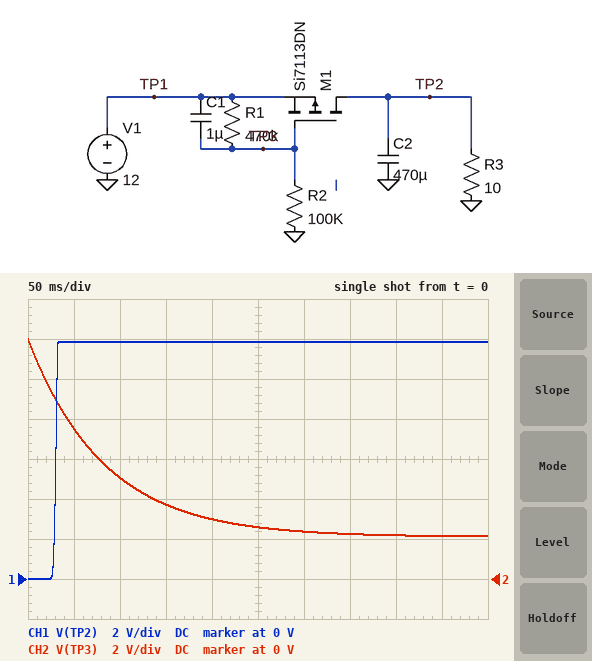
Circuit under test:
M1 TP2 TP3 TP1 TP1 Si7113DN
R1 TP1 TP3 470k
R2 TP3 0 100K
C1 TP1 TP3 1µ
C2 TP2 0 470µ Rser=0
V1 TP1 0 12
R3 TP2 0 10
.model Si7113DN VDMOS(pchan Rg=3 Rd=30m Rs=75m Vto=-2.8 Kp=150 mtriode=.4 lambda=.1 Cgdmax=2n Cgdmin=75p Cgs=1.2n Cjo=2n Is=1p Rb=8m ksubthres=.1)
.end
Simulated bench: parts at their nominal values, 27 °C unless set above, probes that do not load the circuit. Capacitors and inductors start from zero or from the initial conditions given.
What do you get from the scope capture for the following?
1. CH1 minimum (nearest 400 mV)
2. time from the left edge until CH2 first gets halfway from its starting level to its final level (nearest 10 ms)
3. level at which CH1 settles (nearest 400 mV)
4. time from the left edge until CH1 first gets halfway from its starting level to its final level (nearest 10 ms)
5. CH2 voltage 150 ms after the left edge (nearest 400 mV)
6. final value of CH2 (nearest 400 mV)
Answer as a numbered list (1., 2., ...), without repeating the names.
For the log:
1. 0 V
2. 60 ms
3. 12.0 V
4. 30 ms
5. 3.6 V
6. 2.0 V
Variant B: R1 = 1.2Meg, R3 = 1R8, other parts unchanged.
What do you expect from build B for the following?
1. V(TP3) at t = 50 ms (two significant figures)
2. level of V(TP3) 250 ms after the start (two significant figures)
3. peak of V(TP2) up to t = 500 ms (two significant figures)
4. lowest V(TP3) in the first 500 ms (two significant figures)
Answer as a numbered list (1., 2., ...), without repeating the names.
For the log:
1. 7.4 V
2. 1.7 V
3. 11 V
4. 970 mV
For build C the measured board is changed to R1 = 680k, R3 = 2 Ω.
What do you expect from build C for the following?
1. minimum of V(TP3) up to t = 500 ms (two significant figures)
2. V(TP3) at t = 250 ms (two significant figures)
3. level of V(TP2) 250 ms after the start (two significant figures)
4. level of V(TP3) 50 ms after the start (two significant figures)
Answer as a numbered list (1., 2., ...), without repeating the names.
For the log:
1. 1.6 V
2. 2.1 V
3. 11 V
4. 7.4 V
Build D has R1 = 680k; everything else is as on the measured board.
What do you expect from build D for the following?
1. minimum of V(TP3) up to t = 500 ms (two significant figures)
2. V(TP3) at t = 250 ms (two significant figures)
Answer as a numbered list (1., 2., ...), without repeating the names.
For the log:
1. 1.6 V
2. 2.1 V
